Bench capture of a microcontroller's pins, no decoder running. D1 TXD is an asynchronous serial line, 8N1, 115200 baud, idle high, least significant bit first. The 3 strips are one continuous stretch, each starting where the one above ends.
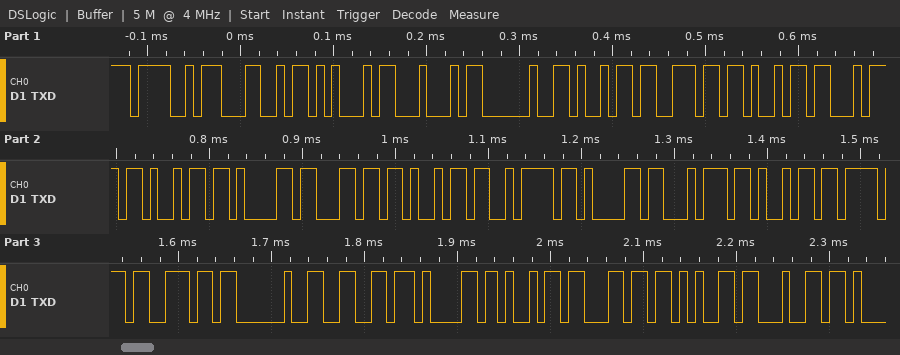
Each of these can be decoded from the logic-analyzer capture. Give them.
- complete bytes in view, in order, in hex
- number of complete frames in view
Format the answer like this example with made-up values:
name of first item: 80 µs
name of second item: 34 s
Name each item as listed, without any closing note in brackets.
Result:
complete bytes in view, in order, in hex: 4F 4C 45 44 20 69 6E 69 74 69 61 6C 69 7A 61 74 69 6F 6E 20 66 61 69 6C 65 64
number of complete frames in view: 26
